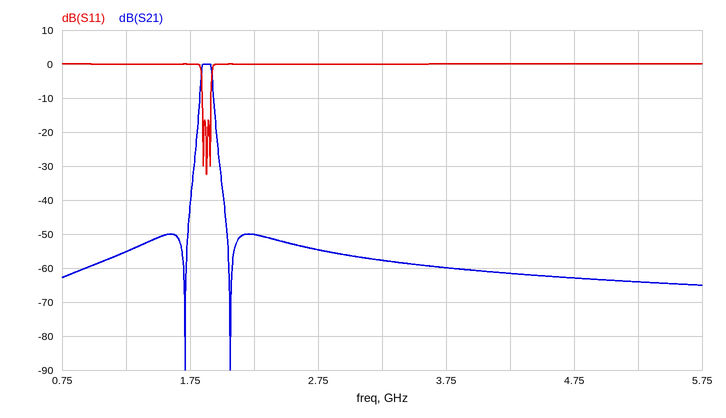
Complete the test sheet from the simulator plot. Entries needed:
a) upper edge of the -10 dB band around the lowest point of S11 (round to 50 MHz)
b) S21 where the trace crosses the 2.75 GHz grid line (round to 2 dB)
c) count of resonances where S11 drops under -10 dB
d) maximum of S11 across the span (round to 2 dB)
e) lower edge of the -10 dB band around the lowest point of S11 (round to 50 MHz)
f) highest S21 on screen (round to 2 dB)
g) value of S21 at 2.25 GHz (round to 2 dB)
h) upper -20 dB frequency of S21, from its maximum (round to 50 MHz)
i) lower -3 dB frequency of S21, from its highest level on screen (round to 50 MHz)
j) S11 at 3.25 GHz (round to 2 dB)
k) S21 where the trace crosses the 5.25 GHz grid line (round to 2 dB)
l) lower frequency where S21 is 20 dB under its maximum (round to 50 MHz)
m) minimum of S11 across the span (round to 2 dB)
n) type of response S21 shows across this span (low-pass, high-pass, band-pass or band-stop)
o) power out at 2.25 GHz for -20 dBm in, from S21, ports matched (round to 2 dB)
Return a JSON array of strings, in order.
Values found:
["1.90 GHz", "-54 dB", "3", "0 dB", "1.85 GHz", "0 dB", "-50 dB", "1.95 GHz", "1.85 GHz", "0 dB", "-64 dB", "1.80 GHz", "-32 dB", "band-pass", "-70 dBm"]
